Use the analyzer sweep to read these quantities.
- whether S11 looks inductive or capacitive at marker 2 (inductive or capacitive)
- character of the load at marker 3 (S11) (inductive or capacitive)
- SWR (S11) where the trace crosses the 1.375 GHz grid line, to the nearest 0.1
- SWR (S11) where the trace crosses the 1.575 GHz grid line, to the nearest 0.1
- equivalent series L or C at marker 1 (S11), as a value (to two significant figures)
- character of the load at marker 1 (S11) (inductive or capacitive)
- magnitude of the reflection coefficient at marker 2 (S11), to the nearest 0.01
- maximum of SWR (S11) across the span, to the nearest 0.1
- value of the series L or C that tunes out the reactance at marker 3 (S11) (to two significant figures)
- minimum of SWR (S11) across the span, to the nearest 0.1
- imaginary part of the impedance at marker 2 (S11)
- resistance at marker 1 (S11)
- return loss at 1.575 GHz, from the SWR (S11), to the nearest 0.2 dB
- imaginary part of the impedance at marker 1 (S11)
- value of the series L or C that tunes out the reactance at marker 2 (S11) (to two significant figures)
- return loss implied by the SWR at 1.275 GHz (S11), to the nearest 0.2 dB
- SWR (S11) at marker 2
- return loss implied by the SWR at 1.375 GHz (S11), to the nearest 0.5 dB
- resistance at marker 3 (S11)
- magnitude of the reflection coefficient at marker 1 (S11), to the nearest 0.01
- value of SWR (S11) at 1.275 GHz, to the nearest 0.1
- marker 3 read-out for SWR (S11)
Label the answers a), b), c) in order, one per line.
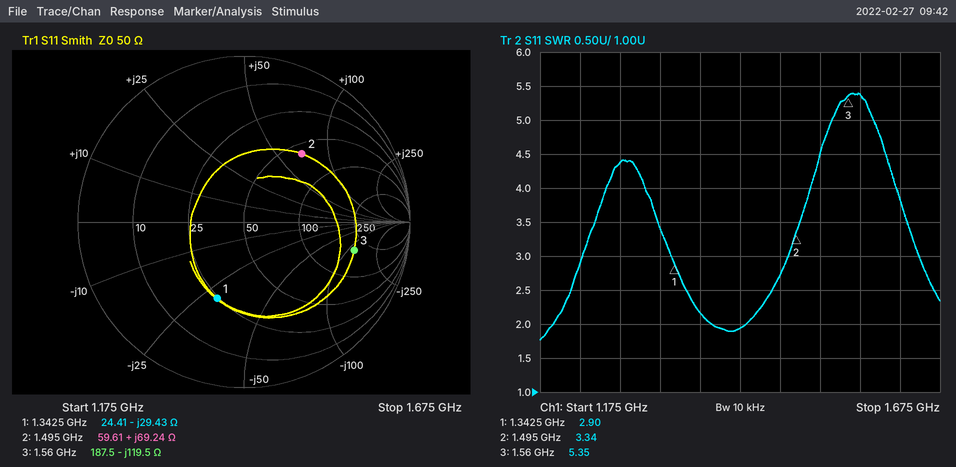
a) inductive
b) capacitive
c) 2.2
d) 5.4
e) 4.0 pF
f) capacitive
g) 0.54
h) 5.4
i) 12 nH
j) 1.8
k) +69.24 Ω
l) 24.41 Ω
m) 3.2 dB
n) -29.43 Ω
o) 1.5 pF
p) 4.0 dB
q) 3.34
r) 8.5 dB
s) 187.5 Ω
t) 0.49
u) 4.4
v) 5.35
